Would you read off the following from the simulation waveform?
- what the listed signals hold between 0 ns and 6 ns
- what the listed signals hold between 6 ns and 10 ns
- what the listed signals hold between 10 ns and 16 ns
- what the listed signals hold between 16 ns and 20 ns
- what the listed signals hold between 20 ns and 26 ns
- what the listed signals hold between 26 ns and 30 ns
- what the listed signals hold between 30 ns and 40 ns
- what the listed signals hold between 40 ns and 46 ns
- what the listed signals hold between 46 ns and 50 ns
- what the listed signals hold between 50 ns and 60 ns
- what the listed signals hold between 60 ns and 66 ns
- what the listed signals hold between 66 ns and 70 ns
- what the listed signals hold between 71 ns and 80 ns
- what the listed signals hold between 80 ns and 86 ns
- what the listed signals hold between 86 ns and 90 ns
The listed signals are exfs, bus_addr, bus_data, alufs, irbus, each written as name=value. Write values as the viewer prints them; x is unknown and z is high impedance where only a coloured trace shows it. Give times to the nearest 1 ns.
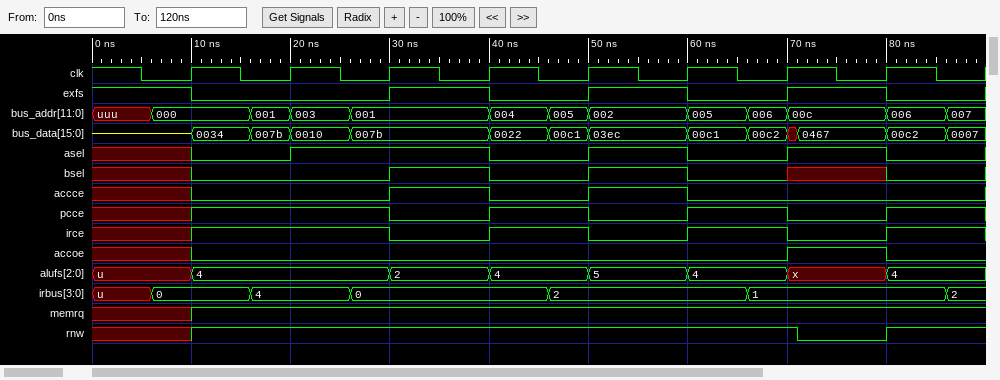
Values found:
exfs=1, bus_addr=uuu, bus_data=z, alufs=u, irbus=u
exfs=1, bus_addr=000, bus_data=z, alufs=u, irbus=0
exfs=0, bus_addr=000, bus_data=0034, alufs=4, irbus=0
exfs=0, bus_addr=001, bus_data=007b, alufs=4, irbus=4
exfs=0, bus_addr=003, bus_data=0010, alufs=4, irbus=4
exfs=0, bus_addr=001, bus_data=007b, alufs=4, irbus=0
exfs=1, bus_addr=001, bus_data=007b, alufs=2, irbus=0
exfs=0, bus_addr=004, bus_data=0022, alufs=4, irbus=0
exfs=0, bus_addr=005, bus_data=00c1, alufs=4, irbus=2
exfs=1, bus_addr=002, bus_data=03ec, alufs=5, irbus=2
exfs=0, bus_addr=005, bus_data=00c1, alufs=4, irbus=2
exfs=0, bus_addr=006, bus_data=00c2, alufs=4, irbus=1
exfs=1, bus_addr=00c, bus_data=0467, alufs=x, irbus=1
exfs=0, bus_addr=006, bus_data=00c2, alufs=4, irbus=1
exfs=0, bus_addr=007, bus_data=0007, alufs=4, irbus=2
